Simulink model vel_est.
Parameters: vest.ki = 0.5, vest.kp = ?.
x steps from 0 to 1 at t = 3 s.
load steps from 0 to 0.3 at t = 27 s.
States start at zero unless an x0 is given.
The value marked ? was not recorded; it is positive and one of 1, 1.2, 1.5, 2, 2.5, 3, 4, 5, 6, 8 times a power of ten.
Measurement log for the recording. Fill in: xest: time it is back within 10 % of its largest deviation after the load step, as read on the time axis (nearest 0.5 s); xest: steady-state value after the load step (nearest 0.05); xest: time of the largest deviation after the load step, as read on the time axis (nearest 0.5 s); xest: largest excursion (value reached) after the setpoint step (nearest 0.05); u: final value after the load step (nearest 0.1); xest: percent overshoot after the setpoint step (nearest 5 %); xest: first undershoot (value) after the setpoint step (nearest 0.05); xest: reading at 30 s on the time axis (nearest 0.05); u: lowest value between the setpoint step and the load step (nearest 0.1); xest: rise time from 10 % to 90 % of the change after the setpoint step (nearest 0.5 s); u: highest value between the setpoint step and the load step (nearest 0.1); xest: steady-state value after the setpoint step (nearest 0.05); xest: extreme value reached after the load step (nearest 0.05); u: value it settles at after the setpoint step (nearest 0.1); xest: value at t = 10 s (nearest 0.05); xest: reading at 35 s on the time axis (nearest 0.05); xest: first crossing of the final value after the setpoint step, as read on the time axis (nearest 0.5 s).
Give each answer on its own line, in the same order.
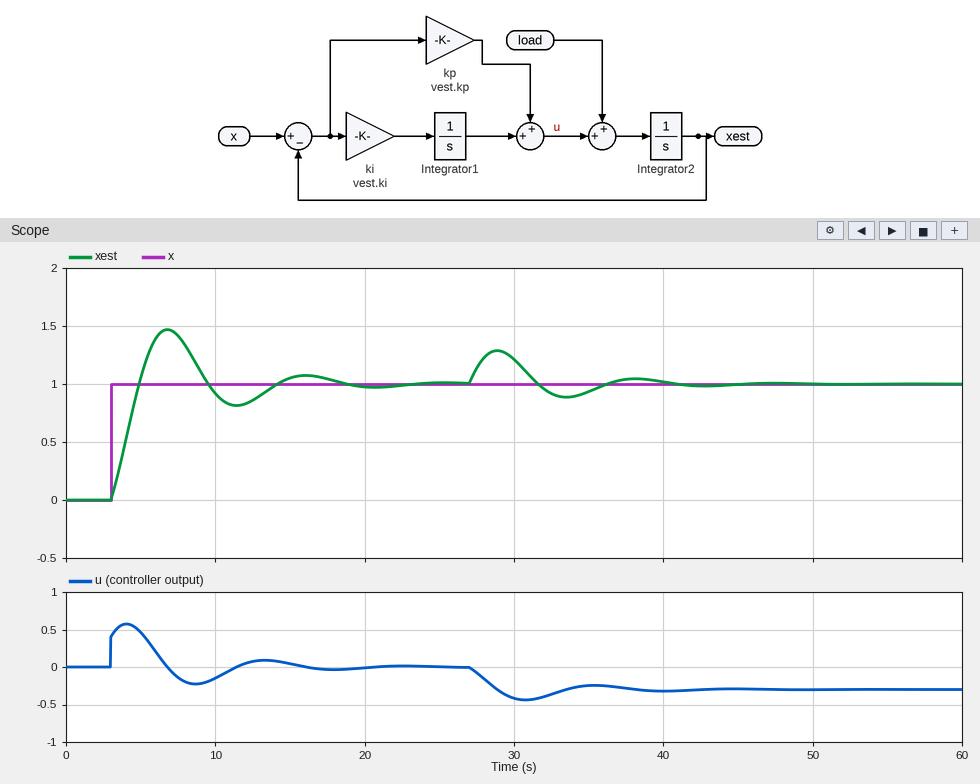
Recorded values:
39.5 s
1.00
29.0 s
1.45
-0.3
45 %
0.80
1.20
-0.2
1.5 s
0.6
1.00
1.30
0.0
0.90
0.95
5.0 s
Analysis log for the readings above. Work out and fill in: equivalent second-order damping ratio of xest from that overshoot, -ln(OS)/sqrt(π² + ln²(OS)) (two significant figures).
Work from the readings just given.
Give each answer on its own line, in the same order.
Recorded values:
0.25
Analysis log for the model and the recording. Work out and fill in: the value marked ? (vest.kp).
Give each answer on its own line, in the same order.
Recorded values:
0.4
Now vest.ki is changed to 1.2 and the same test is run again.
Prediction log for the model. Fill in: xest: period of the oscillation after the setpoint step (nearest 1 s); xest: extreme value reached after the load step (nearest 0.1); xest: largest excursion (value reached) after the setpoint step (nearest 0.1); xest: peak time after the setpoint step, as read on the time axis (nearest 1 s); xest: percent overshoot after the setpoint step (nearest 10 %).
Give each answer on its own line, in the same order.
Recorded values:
6 s
1.2
1.6
6 s
60 %
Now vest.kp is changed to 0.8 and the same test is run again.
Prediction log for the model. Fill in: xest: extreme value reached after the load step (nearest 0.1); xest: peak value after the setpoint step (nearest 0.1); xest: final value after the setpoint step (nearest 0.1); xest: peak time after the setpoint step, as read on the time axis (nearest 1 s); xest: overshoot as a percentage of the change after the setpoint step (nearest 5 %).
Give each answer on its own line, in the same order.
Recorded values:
1.2
1.3
1.0
6 s
25 %
